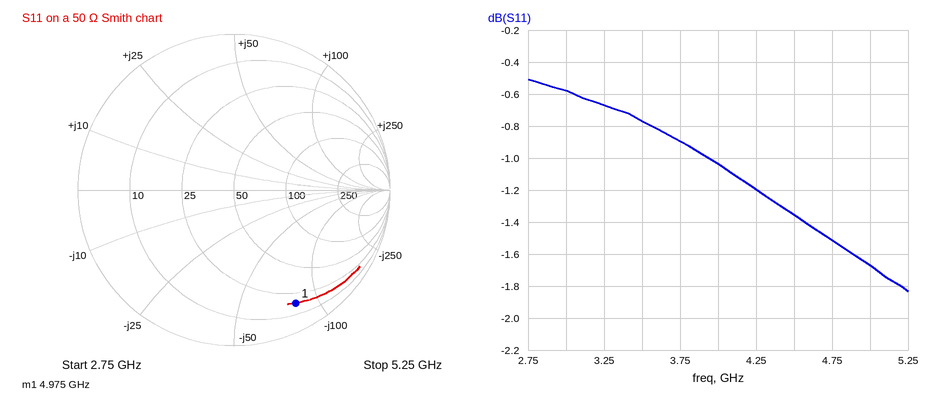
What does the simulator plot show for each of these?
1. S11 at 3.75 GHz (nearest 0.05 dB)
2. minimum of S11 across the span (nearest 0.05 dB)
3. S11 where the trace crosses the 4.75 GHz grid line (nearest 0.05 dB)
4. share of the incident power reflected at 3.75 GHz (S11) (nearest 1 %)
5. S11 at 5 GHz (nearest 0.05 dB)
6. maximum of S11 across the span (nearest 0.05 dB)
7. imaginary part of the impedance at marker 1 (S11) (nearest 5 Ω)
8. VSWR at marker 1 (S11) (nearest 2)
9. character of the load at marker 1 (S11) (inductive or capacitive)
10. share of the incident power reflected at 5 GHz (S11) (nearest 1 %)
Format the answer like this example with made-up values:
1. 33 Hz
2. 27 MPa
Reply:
1. -0.90 dB
2. -1.85 dB
3. -1.50 dB
4. 81 %
5. -1.65 dB
6. -0.50 dB
7. -80 Ω
8. 10
9. capacitive
10. 68 %
